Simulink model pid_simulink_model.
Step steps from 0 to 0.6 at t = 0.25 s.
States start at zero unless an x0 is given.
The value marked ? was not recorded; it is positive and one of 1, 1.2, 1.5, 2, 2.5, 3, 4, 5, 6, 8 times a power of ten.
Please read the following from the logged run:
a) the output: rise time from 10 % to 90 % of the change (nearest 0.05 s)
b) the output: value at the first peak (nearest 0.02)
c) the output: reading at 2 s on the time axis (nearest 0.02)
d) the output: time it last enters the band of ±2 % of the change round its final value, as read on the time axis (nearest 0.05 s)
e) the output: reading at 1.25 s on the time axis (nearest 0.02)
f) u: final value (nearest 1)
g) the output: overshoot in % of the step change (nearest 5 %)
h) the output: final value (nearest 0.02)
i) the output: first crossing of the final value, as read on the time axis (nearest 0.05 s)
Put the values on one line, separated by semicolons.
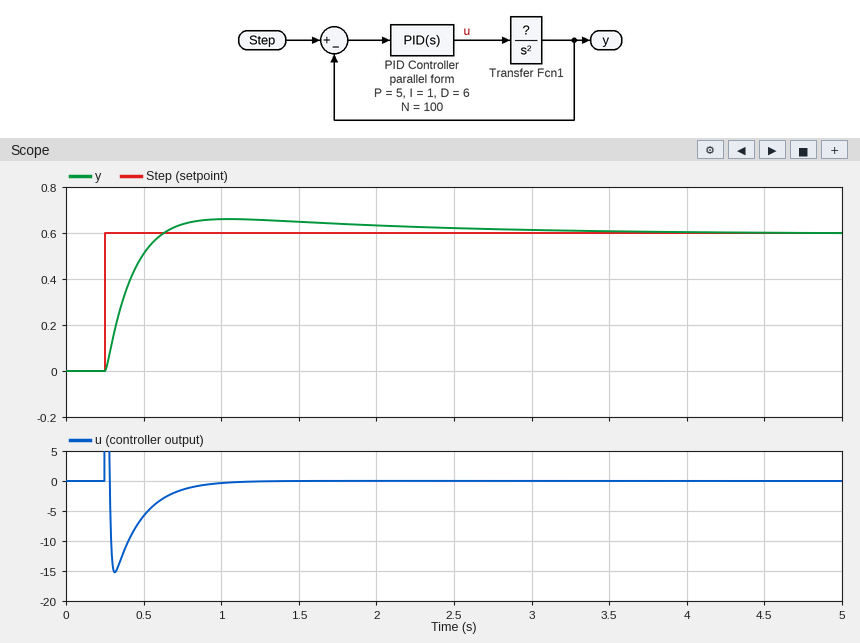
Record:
0.25 s; 0.66; 0.64; 3.10 s; 0.66; 0; 10 %; 0.60; 0.65 s
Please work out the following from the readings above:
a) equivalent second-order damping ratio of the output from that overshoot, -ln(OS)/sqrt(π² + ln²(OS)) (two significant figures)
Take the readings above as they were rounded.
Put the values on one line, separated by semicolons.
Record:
0.59
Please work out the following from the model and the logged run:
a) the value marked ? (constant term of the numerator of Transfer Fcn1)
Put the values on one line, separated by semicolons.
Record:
1
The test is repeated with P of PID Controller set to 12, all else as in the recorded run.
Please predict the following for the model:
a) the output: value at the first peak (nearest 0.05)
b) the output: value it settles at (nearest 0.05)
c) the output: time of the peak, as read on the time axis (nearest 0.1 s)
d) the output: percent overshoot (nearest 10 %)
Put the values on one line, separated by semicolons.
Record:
0.70; 0.60; 0.8 s; 20 %
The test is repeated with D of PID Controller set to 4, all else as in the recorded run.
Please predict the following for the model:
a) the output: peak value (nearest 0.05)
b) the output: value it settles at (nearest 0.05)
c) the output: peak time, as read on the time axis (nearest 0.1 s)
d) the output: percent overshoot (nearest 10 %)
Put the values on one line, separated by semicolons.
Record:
0.70; 0.60; 1.2 s; 20 %
